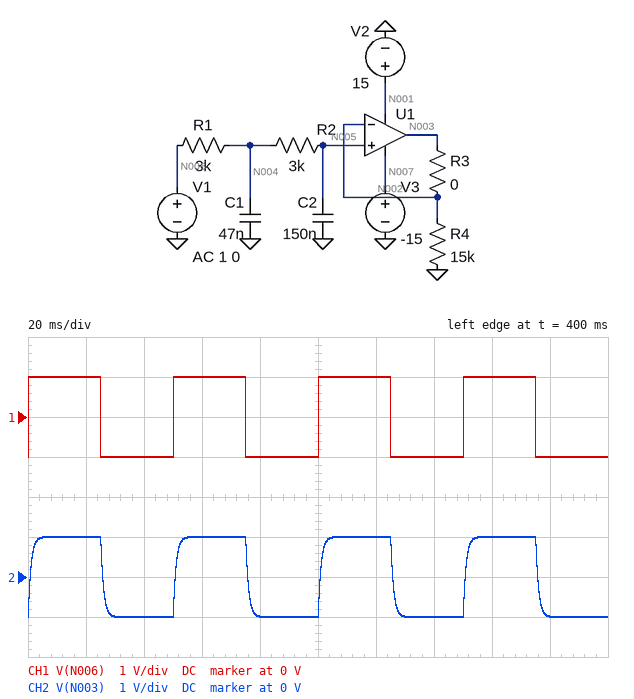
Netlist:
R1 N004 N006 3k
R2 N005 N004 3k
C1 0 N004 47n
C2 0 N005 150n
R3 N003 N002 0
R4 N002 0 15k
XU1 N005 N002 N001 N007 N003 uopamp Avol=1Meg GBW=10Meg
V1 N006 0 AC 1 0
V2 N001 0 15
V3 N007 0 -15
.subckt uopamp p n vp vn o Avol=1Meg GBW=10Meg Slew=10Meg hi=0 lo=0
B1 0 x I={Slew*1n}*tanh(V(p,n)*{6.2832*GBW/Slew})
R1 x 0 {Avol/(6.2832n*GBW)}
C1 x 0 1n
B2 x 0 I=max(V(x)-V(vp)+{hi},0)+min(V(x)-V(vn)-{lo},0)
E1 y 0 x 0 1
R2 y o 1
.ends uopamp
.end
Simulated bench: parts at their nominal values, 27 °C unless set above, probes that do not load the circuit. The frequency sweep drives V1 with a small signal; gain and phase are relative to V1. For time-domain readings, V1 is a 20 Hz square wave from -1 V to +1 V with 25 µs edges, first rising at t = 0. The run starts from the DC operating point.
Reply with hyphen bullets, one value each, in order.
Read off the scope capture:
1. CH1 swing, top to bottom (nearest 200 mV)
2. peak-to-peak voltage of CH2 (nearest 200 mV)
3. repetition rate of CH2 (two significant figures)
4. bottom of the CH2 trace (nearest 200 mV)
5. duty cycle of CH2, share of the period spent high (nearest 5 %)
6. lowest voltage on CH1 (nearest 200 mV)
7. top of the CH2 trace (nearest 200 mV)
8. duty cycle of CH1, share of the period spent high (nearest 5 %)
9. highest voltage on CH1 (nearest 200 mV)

- 2.0 V
- 2.0 V
- 20 Hz
- -1.0 V
- 50 %
- -1.0 V
- 1.0 V
- 50 %
- 1.0 V
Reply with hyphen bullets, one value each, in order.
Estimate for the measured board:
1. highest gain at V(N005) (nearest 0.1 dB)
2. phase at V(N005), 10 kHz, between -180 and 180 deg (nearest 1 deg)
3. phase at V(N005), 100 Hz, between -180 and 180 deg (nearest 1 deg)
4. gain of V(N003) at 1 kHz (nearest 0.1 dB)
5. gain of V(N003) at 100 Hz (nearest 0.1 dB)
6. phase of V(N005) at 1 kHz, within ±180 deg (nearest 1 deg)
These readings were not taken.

- 0 dB
- -165 deg
- -34 deg
- -16.5 dB
- -1.4 dB
- -103 deg
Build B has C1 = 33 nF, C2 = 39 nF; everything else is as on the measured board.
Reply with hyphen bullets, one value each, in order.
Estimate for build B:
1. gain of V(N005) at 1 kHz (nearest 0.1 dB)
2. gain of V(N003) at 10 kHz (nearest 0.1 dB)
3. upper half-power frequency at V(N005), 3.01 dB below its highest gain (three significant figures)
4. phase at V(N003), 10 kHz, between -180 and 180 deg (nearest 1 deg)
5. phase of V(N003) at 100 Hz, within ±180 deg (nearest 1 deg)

- -6.7 dB
- -33.9 dB
- 533 Hz
- -155 deg
- -12 deg
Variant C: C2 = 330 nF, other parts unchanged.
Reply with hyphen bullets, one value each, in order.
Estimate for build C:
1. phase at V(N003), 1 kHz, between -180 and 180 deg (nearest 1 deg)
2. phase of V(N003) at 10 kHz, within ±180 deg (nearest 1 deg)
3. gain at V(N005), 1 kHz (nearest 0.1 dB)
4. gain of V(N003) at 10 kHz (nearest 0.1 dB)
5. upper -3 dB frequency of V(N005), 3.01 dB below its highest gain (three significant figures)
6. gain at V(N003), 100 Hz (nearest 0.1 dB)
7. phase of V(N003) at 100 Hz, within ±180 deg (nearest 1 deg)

- -109 deg
- -166 deg
- -23.0 dB
- -55.1 dB
- 77.4 Hz
- -4.3 dB
- -55 deg
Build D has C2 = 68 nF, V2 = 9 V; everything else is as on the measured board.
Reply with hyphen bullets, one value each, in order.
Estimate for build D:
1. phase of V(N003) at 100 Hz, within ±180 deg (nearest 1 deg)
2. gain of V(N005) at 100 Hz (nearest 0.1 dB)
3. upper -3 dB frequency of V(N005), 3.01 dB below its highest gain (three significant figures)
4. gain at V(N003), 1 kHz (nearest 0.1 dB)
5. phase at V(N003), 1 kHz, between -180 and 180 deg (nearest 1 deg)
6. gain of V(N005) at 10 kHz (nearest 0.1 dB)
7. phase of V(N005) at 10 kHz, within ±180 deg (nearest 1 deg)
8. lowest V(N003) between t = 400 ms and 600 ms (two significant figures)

- -19 deg
- -0.4 dB
- 320 Hz
- -10.8 dB
- -92 deg
- -41.4 dB
- -163 deg
- -1.0 V
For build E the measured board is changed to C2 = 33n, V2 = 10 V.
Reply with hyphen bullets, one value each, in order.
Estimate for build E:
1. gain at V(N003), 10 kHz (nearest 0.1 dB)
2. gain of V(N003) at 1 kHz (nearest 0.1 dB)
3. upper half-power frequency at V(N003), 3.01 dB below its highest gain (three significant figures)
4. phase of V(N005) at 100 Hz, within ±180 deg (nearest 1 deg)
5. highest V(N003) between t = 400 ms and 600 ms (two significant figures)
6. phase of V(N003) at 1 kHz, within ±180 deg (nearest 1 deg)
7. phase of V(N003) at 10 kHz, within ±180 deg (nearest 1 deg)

- -35.3 dB
- -6.8 dB
- 533 Hz
- -12 deg
- 1.0 V
- -78 deg
- -159 deg
